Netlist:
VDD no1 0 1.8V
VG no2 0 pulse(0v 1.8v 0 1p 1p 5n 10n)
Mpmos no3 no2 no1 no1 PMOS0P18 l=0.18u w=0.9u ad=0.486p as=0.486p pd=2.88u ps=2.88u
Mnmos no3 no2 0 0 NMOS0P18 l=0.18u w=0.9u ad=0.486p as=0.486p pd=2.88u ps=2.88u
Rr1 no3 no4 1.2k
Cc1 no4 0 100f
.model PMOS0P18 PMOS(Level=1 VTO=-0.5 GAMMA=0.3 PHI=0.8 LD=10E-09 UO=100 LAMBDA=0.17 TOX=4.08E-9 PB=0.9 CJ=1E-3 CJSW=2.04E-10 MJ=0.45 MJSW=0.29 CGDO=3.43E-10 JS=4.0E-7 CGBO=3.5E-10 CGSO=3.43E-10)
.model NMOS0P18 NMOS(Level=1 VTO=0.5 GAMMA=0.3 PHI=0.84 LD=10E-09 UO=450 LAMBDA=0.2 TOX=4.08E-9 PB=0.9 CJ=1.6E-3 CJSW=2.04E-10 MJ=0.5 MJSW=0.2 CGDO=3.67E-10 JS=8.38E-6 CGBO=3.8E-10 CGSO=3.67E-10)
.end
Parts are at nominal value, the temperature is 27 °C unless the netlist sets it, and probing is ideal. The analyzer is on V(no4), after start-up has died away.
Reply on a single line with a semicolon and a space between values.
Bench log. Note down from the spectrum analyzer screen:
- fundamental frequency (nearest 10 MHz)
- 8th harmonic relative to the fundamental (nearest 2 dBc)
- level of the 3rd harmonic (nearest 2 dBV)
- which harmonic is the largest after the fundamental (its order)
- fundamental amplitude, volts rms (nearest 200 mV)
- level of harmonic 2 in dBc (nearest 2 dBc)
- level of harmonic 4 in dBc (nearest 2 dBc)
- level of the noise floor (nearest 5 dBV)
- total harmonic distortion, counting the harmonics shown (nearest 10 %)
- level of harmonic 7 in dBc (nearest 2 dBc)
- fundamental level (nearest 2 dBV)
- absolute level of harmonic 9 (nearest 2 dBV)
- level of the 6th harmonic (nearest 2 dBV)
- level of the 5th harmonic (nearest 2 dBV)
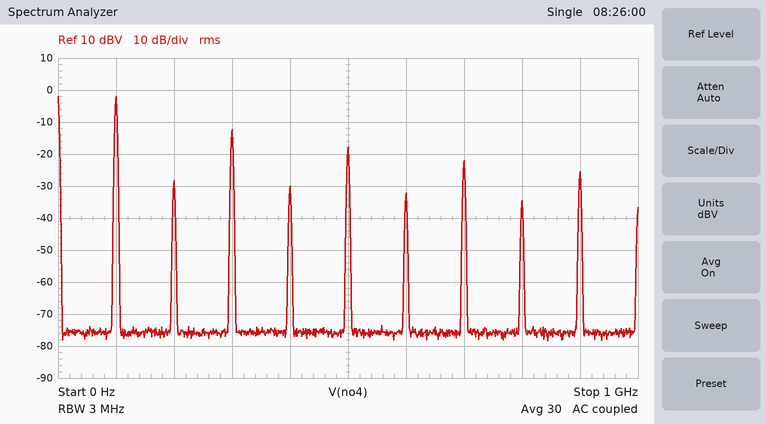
100 MHz; -32 dBc; -12 dBV; 3; 800 mV; -26 dBc; -28 dBc; -75 dBV; 40 %; -20 dBc; -2 dBV; -26 dBV; -32 dBV; -18 dBV
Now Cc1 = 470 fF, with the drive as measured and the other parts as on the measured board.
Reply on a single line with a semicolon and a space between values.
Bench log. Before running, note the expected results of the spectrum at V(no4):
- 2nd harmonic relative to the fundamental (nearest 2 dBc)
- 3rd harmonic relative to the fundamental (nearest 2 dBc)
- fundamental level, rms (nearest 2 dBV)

-20 dBc; -14 dBc; -4 dBV
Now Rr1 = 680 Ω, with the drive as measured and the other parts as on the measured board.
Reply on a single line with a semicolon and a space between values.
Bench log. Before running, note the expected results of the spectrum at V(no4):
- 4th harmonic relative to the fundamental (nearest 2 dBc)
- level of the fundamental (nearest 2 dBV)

-26 dBc; -2 dBV
